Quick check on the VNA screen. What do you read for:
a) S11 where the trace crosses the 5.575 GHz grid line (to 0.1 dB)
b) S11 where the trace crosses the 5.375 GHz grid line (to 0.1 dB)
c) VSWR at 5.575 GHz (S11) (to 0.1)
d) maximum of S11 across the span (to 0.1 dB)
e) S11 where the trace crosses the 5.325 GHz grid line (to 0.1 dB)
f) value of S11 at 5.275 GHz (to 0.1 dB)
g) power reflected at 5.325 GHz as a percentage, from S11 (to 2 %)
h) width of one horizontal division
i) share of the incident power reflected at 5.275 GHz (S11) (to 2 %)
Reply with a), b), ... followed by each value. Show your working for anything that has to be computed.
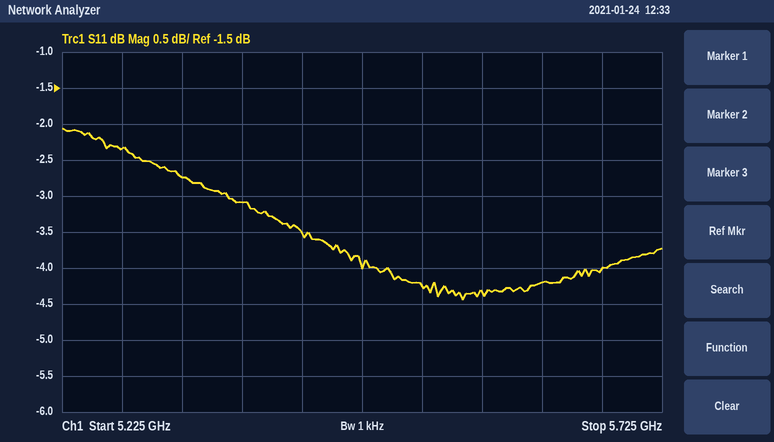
a) -4.3 dB
b) -3.1 dB
c) |Γ| = 10^(-4.3/20) = 0.6095; VSWR = (1 + 0.6095)/(1 − 0.6095) ≈ 4.1
d) -2.1 dB
e) -2.7 dB
f) -2.3 dB
g) 10^(-2.7/10) ≈ 54 %
h) 50 MHz
i) 10^(-2.3/10) ≈ 58.9 %, so 58 % to the nearest 2 %
